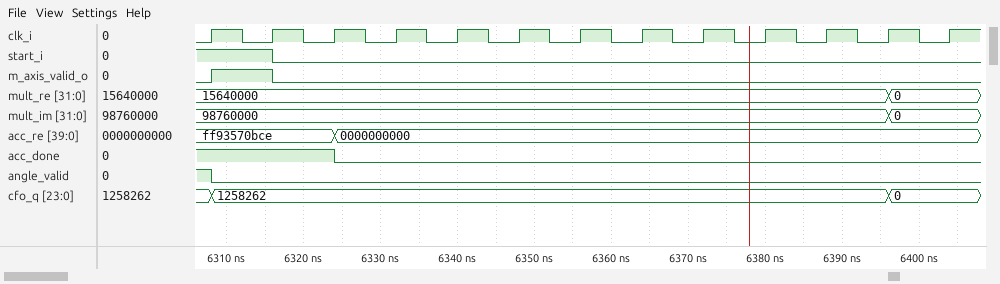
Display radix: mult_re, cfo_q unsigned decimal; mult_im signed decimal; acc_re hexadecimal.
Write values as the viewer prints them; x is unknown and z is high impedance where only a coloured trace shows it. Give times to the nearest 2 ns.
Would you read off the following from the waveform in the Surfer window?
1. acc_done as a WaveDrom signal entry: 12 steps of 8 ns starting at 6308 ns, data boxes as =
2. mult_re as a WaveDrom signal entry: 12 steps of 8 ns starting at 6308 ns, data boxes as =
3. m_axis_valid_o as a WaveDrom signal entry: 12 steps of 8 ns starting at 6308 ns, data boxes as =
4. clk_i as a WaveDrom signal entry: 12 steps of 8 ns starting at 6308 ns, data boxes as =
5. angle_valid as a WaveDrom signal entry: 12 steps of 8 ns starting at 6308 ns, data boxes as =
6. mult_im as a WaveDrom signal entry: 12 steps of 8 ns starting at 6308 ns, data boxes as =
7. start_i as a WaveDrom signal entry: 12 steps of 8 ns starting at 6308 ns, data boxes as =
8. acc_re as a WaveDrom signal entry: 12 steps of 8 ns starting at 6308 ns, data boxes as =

{name: 'acc_done', wave: '1.0.........'}
{name: 'mult_re', wave: '=..........=', data: '15640000 0'}
{name: 'm_axis_valid_o', wave: '10..........'}
{name: 'clk_i', wave: 'p...........'}
{name: 'angle_valid', wave: '0...........'}
{name: 'mult_im', wave: '=..........=', data: '98760000 0'}
{name: 'start_i', wave: '10..........'}
{name: 'acc_re', wave: '=.=.........', data: 'ff93570bce 0000000000'}
